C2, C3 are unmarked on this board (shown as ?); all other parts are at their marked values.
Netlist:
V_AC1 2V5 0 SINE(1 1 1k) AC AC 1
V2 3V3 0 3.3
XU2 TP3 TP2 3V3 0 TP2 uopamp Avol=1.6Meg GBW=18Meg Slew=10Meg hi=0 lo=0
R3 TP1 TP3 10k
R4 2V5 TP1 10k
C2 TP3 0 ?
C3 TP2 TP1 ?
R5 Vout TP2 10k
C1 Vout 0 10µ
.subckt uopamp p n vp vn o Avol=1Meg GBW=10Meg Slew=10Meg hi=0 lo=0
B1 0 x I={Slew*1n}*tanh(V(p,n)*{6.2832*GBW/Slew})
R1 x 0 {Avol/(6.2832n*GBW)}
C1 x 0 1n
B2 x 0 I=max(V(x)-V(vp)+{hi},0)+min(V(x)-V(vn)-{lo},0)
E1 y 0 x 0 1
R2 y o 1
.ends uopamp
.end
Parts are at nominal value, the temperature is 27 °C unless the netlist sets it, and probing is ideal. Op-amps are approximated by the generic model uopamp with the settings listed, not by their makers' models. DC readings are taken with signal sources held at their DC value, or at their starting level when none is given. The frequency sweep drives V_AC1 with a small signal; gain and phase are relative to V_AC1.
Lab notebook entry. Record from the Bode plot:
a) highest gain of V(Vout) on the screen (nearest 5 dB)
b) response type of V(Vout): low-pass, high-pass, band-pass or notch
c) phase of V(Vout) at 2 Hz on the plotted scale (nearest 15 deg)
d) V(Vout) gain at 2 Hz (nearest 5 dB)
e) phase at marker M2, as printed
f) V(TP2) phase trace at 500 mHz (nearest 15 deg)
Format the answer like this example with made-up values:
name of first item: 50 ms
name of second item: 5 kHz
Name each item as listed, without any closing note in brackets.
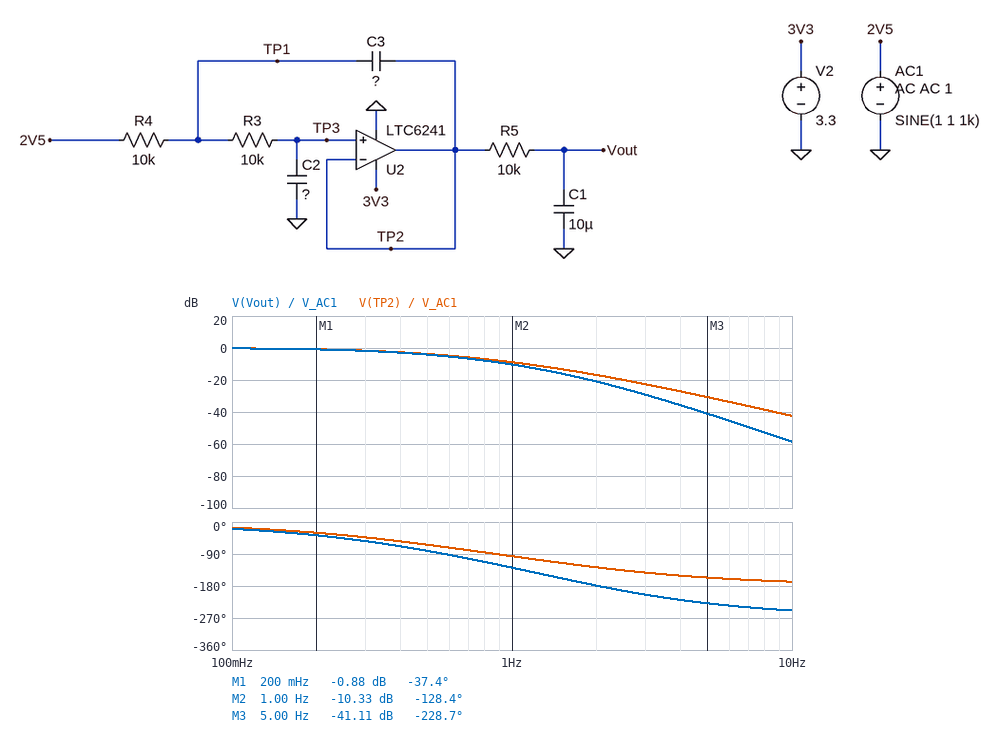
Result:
highest gain of V(Vout) on the screen: 0 dB
response type of V(Vout): low-pass, high-pass, band-pass or notch: low-pass
phase of V(Vout) at 2 Hz on the plotted scale: -180 deg
V(Vout) gain at 2 Hz: -20 dB
phase at marker M2, as printed: -128.4 deg
V(TP2) phase trace at 500 mHz: -60 deg
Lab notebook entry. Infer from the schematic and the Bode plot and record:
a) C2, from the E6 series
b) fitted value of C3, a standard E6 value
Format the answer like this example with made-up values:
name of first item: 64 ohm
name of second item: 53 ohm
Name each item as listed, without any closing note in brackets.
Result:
C2, from the E6 series: 22 µF
fitted value of C3, a standard E6 value: 15 µF
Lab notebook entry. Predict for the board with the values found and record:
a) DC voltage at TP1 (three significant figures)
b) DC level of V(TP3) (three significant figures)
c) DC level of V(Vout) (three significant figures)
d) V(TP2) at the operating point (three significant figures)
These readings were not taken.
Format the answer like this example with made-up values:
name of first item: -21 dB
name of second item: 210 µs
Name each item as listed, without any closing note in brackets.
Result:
DC voltage at TP1: 1.00 V
DC level of V(TP3): 1.00 V
DC level of V(Vout): 1.00 V
V(TP2) at the operating point: 1.00 V
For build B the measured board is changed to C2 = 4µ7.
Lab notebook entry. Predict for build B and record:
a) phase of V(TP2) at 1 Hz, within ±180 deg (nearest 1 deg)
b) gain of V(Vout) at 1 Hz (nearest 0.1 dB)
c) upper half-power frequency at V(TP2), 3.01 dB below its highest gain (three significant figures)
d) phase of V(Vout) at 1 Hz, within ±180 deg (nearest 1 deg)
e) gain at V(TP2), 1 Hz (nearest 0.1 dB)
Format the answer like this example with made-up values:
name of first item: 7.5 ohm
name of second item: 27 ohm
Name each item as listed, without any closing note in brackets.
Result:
phase of V(TP2) at 1 Hz, within ±180 deg: -39 deg
gain of V(Vout) at 1 Hz: -0.8 dB
upper half-power frequency at V(TP2), 3.01 dB below its highest gain: 2.16 Hz
phase of V(Vout) at 1 Hz, within ±180 deg: -71 deg
gain at V(TP2), 1 Hz: 0.6 dB
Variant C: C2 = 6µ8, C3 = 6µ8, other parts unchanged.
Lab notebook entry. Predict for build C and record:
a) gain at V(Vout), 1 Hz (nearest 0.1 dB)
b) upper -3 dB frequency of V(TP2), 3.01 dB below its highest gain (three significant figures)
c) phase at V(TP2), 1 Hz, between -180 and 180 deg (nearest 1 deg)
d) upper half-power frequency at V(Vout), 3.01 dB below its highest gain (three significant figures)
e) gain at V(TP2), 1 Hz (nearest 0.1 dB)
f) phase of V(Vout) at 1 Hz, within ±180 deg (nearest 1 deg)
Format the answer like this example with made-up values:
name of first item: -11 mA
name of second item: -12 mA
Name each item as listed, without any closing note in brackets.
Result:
gain at V(Vout), 1 Hz: -2.9 dB
upper -3 dB frequency of V(TP2), 3.01 dB below its highest gain: 1.51 Hz
phase at V(TP2), 1 Hz, between -180 and 180 deg: -46 deg
upper half-power frequency at V(Vout), 3.01 dB below its highest gain: 1.02 Hz
gain at V(TP2), 1 Hz: -1.5 dB
phase of V(Vout) at 1 Hz, within ±180 deg: -78 deg
